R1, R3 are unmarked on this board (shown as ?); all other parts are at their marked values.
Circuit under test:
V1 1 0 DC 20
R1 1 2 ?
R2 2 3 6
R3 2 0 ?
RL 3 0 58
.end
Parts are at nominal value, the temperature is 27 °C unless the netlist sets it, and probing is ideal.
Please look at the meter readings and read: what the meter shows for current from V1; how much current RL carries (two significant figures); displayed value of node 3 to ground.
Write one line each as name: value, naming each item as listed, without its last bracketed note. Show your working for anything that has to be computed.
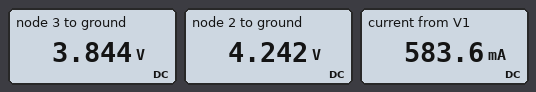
what the meter shows for current from V1: 583.6 mA
how much current RL carries: (3.844 V) / 58 Ω = 66 mA
displayed value of node 3 to ground: 3.844 V
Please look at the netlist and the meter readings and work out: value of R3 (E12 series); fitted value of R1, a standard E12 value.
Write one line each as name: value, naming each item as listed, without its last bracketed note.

value of R3: 8.2 Ω
fitted value of R1, a standard E12 value: 27 Ω
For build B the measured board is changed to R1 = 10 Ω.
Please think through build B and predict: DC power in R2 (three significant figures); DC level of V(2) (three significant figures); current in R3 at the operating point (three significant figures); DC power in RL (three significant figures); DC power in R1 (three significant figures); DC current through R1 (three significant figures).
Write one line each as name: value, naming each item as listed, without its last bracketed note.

DC power in R2: 104 mW
DC level of V(2): 8.42 V
current in R3 at the operating point: 1.03 A
DC power in RL: 1.00 W
DC power in R1: 13.4 W
DC current through R1: 1.16 A
